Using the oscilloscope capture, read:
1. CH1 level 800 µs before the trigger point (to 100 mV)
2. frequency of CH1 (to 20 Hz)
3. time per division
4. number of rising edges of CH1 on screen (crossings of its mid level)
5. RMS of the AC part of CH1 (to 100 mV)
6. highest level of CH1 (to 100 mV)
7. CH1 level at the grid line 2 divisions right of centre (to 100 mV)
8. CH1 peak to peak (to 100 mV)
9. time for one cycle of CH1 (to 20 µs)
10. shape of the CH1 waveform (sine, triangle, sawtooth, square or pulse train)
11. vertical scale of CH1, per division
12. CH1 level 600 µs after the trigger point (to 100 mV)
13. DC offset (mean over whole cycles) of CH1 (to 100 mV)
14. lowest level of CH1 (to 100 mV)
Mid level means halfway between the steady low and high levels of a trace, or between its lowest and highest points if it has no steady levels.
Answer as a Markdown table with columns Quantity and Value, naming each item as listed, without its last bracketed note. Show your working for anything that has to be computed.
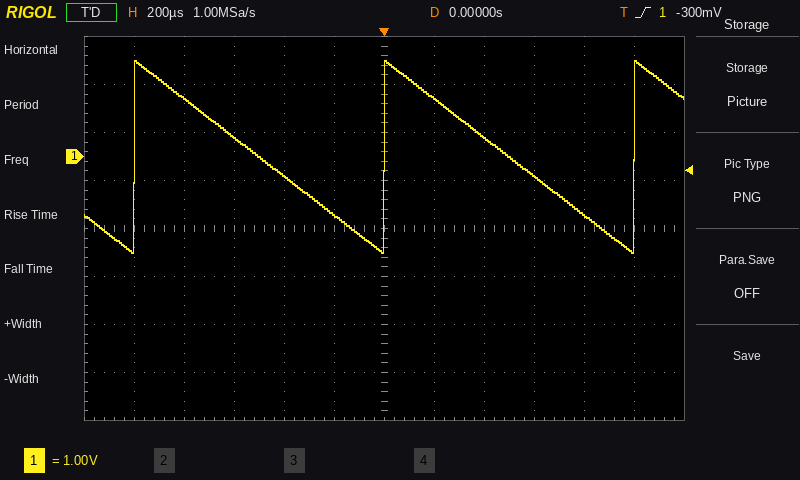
| Quantity | Value |
|---|---|
| CH1 level 800 µs before the trigger point | 1.2 V |
| frequency of CH1 | 1 / 1.00 ms ≈ 1.00 kHz |
| time per division | 200 µs |
| number of rising edges of CH1 on screen | 3 |
| RMS of the AC part of CH1 | 4.0 V / (2√3) ≈ 1.2 V |
| highest level of CH1 | 2.0 V |
| CH1 level at the grid line 2 divisions right of centre | 400 mV |
| CH1 peak to peak | 2.0 V − (-2.0 V) = 4.0 V |
| time for one cycle of CH1 | 1.00 ms |
| shape of the CH1 waveform | sawtooth |
| vertical scale of CH1, per division | 1 V |
| CH1 level 600 µs after the trigger point | -400 mV |
| DC offset (mean over whole cycles) of CH1 | (2.0 V + (-2.0 V)) / 2 ≈ 0.0 V |
| lowest level of CH1 | -2.0 V |
